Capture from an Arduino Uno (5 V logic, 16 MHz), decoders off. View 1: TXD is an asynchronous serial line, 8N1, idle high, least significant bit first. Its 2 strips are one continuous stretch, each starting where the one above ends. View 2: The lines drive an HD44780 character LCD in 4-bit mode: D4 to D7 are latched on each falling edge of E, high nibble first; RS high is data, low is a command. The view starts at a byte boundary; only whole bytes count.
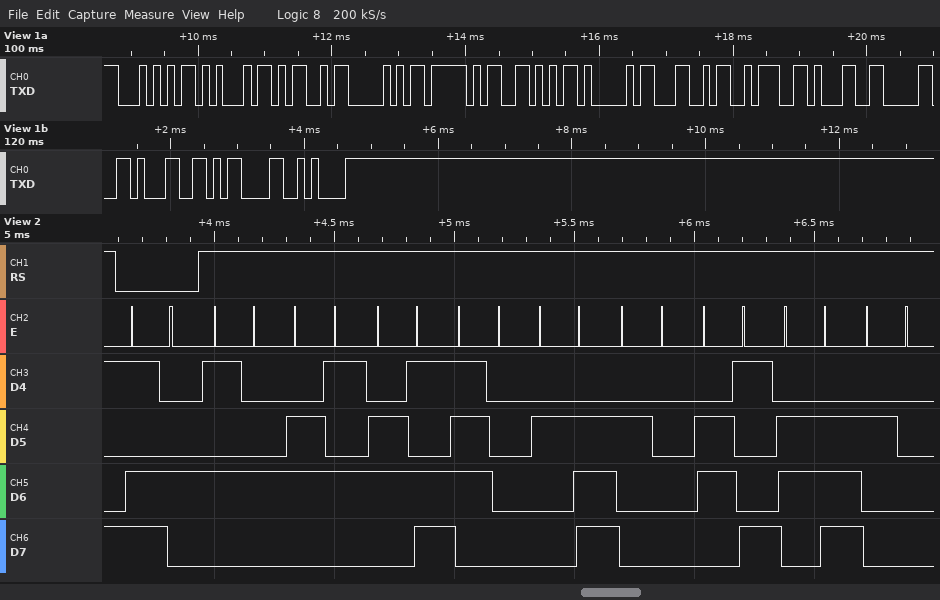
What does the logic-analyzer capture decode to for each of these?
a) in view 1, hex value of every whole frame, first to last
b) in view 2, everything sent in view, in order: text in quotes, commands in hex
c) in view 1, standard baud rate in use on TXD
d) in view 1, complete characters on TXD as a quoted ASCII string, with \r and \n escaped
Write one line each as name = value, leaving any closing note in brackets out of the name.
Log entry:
in view 1, hex value of every whole frame, first to last = 54 45 4D 50 5F 56 41 4C 3A 31 30 31 0D 0A
in view 2, everything sent in view, in order: text in quotes, commands in hex = 0xD4 "Temp. in "
in view 1, standard baud rate in use on TXD = 9600 baud
in view 1, complete characters on TXD as a quoted ASCII string, with \r and \n escaped = "TEMP_VAL:101\r\n"
